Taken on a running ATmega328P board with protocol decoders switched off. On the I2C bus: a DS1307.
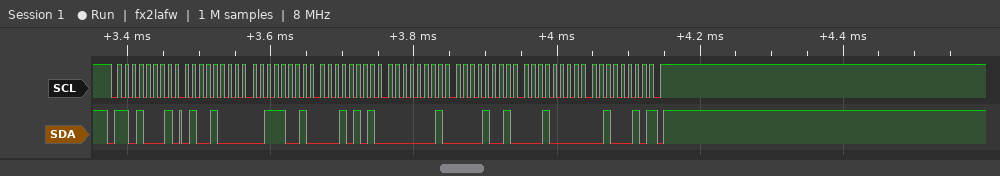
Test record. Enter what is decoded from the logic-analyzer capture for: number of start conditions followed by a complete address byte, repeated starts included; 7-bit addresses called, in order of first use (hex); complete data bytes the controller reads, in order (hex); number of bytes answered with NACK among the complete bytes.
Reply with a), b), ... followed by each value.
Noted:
a) 1
b) 0x68
c) 48 39 15 01 09 10 22
d) 1
